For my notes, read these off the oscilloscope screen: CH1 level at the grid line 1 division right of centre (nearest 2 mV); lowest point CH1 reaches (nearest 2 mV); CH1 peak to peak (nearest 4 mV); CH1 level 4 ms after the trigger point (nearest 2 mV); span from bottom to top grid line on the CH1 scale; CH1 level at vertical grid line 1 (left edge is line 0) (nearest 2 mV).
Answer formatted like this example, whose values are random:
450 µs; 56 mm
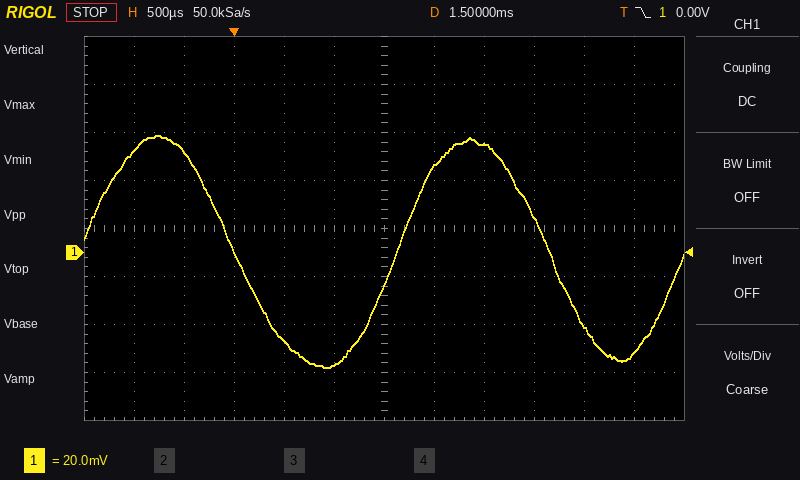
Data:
36 mV; -48 mV; 96 mV; -42 mV; 160 mV; 42 mV
